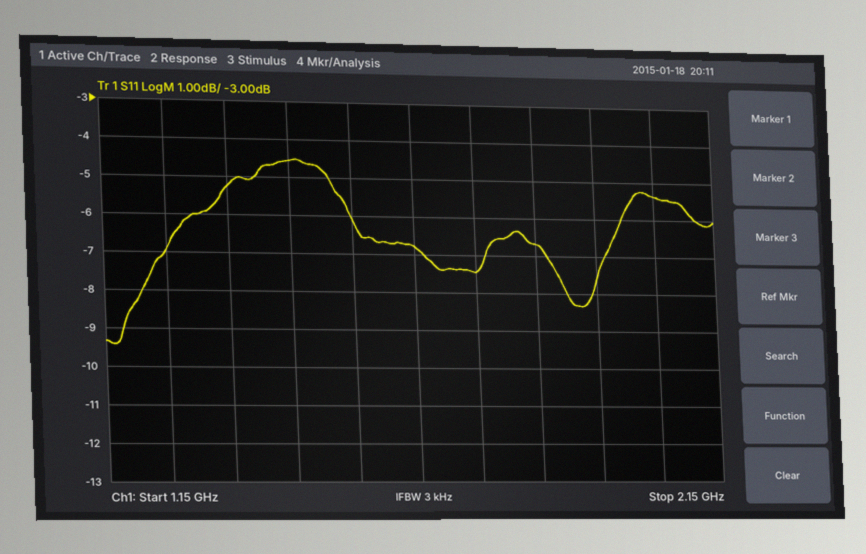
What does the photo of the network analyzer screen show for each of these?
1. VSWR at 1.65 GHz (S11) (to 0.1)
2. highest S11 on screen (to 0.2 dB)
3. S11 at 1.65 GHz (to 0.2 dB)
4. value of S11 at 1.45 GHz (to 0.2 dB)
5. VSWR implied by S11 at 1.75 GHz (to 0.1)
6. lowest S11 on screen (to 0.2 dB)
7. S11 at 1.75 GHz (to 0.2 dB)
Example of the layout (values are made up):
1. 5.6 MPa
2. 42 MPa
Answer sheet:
1. 2.7
2. -4.6 dB
3. -6.8 dB
4. -4.6 dB
5. 2.5
6. -9.4 dB
7. -7.4 dB
